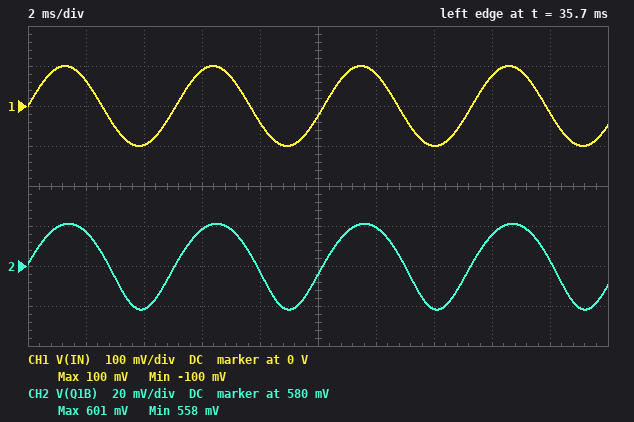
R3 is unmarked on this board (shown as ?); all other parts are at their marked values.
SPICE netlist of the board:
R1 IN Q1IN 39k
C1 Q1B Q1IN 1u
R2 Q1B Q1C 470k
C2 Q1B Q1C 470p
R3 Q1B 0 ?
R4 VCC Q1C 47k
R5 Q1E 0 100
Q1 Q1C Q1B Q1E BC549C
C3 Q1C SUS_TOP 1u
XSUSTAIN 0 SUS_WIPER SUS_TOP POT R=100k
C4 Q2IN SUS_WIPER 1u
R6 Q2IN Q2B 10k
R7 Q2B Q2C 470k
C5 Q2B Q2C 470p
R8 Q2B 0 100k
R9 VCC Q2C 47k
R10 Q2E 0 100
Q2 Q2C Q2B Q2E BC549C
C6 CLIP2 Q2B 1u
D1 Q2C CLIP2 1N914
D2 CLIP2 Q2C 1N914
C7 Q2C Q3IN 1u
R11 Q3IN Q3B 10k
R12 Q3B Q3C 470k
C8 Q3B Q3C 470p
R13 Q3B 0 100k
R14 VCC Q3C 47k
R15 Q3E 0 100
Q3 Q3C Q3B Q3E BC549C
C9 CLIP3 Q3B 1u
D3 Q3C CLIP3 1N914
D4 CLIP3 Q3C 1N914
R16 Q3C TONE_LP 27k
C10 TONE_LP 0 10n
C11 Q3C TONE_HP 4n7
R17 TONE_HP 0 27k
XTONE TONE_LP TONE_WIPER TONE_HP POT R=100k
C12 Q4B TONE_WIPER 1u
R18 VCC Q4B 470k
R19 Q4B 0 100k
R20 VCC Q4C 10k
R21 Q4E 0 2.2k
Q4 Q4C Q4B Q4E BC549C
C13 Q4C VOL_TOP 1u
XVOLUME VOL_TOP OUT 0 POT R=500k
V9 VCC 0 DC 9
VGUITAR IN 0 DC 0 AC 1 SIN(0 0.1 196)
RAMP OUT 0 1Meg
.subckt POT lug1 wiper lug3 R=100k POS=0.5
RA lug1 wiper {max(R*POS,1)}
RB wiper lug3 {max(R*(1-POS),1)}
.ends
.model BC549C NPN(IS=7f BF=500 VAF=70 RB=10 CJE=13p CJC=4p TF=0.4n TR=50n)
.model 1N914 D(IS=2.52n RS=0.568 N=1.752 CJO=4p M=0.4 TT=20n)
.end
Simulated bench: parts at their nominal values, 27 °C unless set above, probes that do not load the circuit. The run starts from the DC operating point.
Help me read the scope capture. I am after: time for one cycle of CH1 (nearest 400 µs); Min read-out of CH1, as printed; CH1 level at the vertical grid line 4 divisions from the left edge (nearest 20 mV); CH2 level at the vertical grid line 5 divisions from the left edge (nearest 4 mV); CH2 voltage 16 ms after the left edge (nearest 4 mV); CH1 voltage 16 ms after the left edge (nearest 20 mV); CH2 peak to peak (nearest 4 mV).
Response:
5.2 ms
-100 mV
-40 mV
576 mV
596 mV
80 mV
44 mV
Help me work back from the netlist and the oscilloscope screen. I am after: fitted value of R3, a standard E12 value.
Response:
47 kΩ
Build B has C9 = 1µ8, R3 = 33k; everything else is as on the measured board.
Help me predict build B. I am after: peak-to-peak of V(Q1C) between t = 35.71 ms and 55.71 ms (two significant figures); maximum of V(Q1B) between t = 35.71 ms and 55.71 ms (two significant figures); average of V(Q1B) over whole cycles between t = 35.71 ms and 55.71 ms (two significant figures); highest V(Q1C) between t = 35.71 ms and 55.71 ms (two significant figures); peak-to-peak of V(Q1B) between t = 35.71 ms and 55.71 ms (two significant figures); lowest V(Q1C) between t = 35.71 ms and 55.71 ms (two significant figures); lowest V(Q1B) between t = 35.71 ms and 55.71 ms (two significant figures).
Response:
380 mV
560 mV
520 mV
8.1 V
74 mV
7.7 V
480 mV
